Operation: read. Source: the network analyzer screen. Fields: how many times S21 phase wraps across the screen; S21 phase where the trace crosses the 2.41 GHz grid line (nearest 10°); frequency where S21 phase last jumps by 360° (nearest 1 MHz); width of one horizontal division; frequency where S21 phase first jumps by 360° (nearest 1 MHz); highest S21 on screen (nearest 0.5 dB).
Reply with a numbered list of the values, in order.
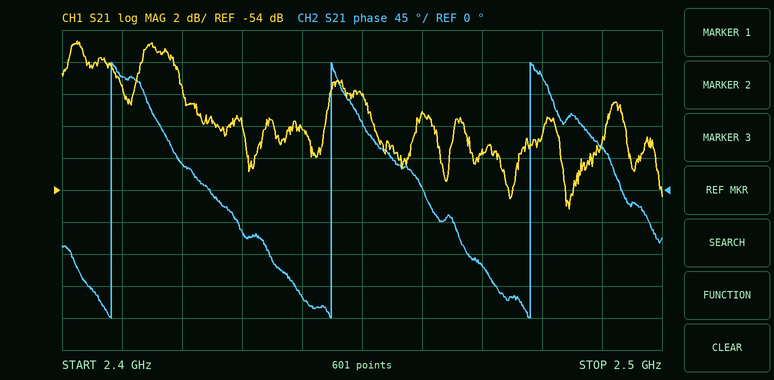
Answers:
1. 3
2. 160°
3. 2.478 GHz
4. 10 MHz
5. 2.408 GHz
6. -44.5 dB
